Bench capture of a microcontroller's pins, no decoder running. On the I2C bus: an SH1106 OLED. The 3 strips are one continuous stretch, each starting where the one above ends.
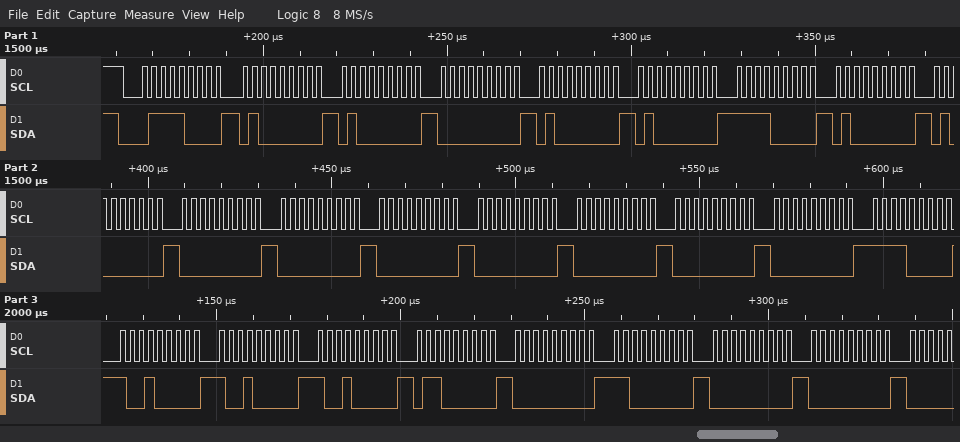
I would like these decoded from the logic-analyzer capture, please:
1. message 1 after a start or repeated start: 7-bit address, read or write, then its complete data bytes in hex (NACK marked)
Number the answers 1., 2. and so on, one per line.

1. 0x3C write: 40 40 00 40 40 F0 40 40 00 00 00 00 00 00 00 F0 90 90 90 60 00 C0 00 00
